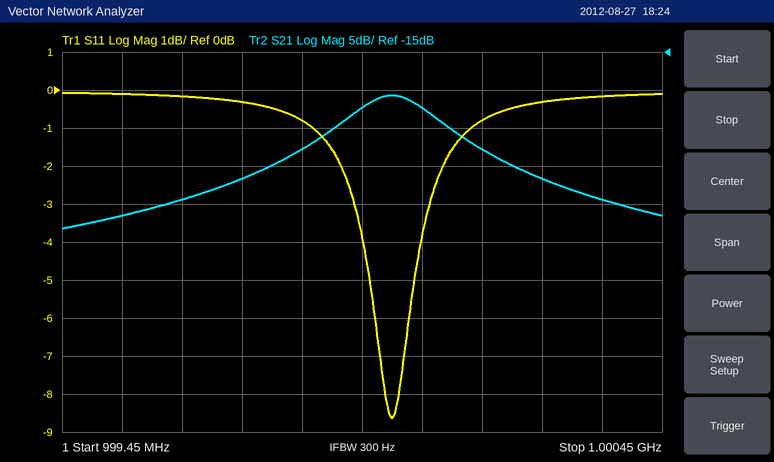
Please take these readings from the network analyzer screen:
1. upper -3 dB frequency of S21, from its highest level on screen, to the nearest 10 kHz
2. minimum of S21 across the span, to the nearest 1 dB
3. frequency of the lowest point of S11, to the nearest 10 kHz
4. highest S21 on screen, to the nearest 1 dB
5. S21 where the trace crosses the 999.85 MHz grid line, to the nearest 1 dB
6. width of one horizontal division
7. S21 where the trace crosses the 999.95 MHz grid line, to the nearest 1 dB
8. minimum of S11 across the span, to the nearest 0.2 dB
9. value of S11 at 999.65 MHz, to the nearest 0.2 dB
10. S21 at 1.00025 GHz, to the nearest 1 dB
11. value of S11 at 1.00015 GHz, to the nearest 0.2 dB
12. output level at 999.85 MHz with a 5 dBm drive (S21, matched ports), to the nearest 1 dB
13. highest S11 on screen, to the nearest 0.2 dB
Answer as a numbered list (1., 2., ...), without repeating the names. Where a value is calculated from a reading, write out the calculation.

1. 1.00007 GHz
2. -38 dB
3. 1.00000 GHz
4. -21 dB
5. -28 dB
6. 100 kHz
7. -22 dB
8. -8.6 dB
9. -0.2 dB
10. -32 dB
11. -0.8 dB
12. 5 dBm + (-28 dB) = -23 dBm
13. 0.0 dB
